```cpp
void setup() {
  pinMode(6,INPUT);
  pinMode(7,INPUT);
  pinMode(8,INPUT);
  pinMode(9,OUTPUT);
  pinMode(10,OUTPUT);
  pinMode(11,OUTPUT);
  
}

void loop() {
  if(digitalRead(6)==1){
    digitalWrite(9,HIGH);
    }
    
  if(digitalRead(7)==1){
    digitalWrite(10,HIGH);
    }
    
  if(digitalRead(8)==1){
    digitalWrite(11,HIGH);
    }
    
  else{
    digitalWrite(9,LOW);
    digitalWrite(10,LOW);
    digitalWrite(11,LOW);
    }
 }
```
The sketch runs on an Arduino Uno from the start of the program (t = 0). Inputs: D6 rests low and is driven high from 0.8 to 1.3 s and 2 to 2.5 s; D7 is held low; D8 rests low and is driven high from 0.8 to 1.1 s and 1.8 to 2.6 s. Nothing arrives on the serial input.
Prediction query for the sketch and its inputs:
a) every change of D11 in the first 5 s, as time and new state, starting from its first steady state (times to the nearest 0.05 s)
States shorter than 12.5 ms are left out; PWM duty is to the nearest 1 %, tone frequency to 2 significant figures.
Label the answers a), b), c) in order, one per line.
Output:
a) 0 s low; 0.8 s high; 1.1 s low; 1.8 s high; 2.6 s low
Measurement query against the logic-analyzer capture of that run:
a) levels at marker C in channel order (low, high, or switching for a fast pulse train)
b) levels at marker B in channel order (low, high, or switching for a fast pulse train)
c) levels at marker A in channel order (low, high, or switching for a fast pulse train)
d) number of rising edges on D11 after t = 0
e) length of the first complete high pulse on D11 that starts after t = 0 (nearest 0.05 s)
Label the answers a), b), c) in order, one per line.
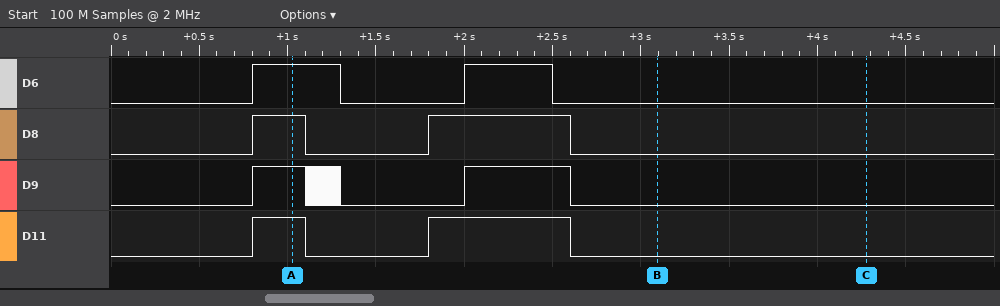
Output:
a) D6 low, D8 low, D9 low, D11 low
b) D6 low, D8 low, D9 low, D11 low
c) D6 high, D8 high, D9 high, D11 high
d) 2
e) 0.30 s
